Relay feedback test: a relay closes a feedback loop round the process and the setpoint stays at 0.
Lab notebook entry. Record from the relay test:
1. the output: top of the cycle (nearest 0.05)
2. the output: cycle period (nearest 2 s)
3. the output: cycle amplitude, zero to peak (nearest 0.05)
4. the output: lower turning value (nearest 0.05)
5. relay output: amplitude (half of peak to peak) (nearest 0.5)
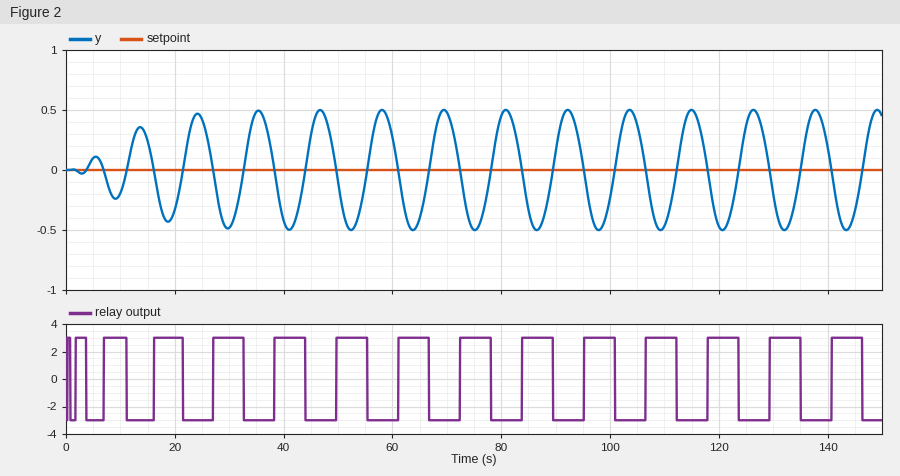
0.50
12 s
0.50
-0.50
3.0
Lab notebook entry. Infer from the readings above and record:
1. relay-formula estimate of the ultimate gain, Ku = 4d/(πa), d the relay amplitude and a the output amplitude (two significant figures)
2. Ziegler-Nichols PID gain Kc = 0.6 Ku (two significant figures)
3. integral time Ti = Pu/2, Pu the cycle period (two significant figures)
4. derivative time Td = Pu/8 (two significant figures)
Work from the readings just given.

7.6
4.6
6.0 s
1.5 s
